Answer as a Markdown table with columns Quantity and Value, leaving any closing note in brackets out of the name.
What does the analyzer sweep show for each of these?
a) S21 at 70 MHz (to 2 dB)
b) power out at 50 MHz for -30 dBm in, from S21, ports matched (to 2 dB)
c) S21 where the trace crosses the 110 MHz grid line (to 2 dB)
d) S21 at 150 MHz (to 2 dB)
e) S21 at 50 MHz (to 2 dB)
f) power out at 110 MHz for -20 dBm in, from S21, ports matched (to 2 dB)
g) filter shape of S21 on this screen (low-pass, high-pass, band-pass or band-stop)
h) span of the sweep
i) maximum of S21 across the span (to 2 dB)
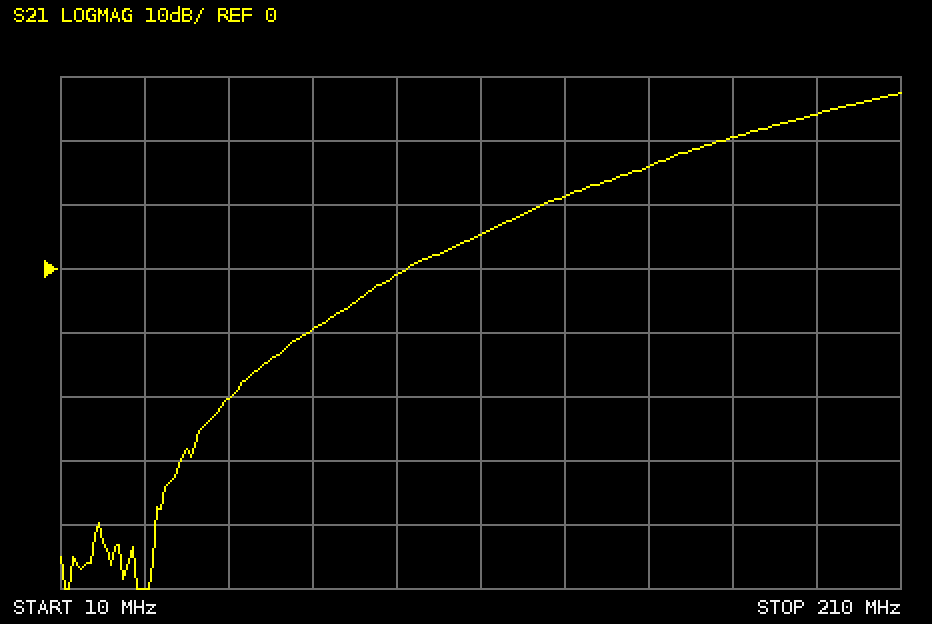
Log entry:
| Quantity | Value |
|---|---|
| S21 at 70 MHz | -10 dB |
| power out at 50 MHz for -30 dBm in, from S21, ports matched | -50 dBm |
| S21 where the trace crosses the 110 MHz grid line | 6 dB |
| S21 at 150 MHz | 16 dB |
| S21 at 50 MHz | -20 dB |
| power out at 110 MHz for -20 dBm in, from S21, ports matched | -14 dBm |
| filter shape of S21 on this screen | high-pass |
| span of the sweep | 200 MHz |
| maximum of S21 across the span | 28 dB |
